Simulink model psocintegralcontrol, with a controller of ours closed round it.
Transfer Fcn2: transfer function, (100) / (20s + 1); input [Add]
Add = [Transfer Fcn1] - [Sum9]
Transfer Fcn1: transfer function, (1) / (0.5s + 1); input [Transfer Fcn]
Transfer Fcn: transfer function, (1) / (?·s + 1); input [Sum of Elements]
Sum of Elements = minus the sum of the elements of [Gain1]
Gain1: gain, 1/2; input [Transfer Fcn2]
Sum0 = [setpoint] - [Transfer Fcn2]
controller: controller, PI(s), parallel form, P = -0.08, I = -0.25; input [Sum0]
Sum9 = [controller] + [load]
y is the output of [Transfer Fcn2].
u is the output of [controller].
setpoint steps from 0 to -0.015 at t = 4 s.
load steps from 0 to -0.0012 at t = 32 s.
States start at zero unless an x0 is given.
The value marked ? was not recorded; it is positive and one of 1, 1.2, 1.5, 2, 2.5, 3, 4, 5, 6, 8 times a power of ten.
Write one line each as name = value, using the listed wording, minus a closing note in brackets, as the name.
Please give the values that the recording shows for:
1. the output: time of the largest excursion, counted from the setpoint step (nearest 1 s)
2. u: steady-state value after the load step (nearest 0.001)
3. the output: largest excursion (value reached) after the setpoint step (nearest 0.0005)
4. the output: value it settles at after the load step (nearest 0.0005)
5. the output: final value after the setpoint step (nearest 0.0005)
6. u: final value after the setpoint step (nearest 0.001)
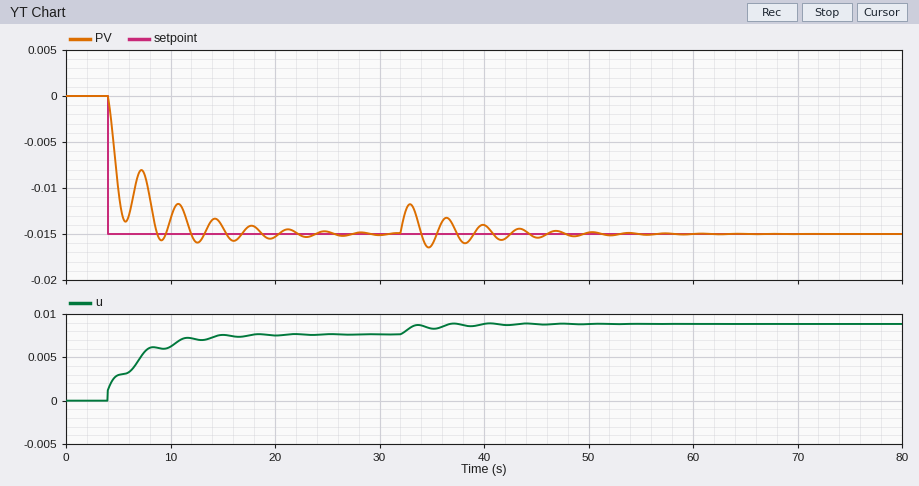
the output: time of the largest excursion, counted from the setpoint step = 9 s
u: steady-state value after the load step = 0.009
the output: largest excursion (value reached) after the setpoint step = -0.0160
the output: value it settles at after the load step = -0.0150
the output: final value after the setpoint step = -0.0150
u: final value after the setpoint step = 0.008
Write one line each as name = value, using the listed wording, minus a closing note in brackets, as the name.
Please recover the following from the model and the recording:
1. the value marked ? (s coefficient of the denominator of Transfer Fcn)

the value marked ? = 0.8
